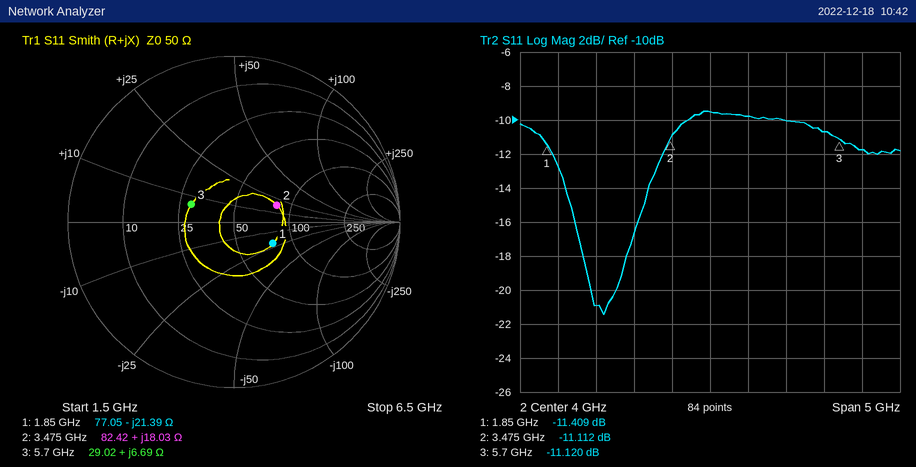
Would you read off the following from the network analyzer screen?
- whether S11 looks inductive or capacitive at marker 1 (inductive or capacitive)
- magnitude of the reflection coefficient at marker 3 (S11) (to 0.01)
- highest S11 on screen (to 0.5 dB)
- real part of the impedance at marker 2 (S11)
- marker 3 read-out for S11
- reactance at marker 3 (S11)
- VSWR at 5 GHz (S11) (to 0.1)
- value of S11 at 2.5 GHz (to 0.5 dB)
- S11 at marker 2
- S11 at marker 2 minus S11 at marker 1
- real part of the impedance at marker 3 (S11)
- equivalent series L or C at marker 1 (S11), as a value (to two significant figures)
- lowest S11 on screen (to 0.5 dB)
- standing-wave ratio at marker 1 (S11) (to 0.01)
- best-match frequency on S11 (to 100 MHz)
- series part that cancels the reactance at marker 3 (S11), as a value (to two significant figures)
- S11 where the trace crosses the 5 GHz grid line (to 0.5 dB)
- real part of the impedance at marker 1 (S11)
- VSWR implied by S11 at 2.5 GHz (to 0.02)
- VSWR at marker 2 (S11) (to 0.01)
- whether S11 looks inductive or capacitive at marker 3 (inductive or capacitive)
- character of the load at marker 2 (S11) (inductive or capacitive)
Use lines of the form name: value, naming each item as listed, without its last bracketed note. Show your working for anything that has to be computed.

whether S11 looks inductive or capacitive at marker 1: capacitive
magnitude of the reflection coefficient at marker 3 (S11): 0.28
highest S11 on screen: -9.5 dB
real part of the impedance at marker 2: 82.42 Ω
marker 3 read-out for S11: -11.120 dB
reactance at marker 3: +6.69 Ω
VSWR at 5 GHz (S11): |Γ| = 10^(-10/20) = 0.3162; VSWR = (1 + 0.3162)/(1 − 0.3162) ≈ 1.9
value of S11 at 2.5 GHz: -21.0 dB
S11 at marker 2: -11.112 dB
S11 at marker 2 minus S11 at marker 1: -11.112 − (-11.409) = 0.297 dB
real part of the impedance at marker 3: 29.02 Ω
equivalent series L or C at marker 1 (S11), as a value: C = 1/(2π × 1.85 GHz × 21.39 Ω) ≈ 4.0 pF
lowest S11 on screen: -21.5 dB
standing-wave ratio at marker 1 (S11): 1.73
best-match frequency on S11: 2.6 GHz
series part that cancels the reactance at marker 3 (S11), as a value: C = 1/(2π × 5.7 GHz × 6.69 Ω) ≈ 4.2 pF
S11 where the trace crosses the 5 GHz grid line: -10.0 dB
real part of the impedance at marker 1: 77.05 Ω
VSWR implied by S11 at 2.5 GHz: |Γ| = 10^(-21/20) = 0.0891; VSWR = (1 + 0.0891)/(1 − 0.0891) ≈ 1.20
VSWR at marker 2 (S11): 1.77
whether S11 looks inductive or capacitive at marker 3: inductive
character of the load at marker 2 (S11): inductive
